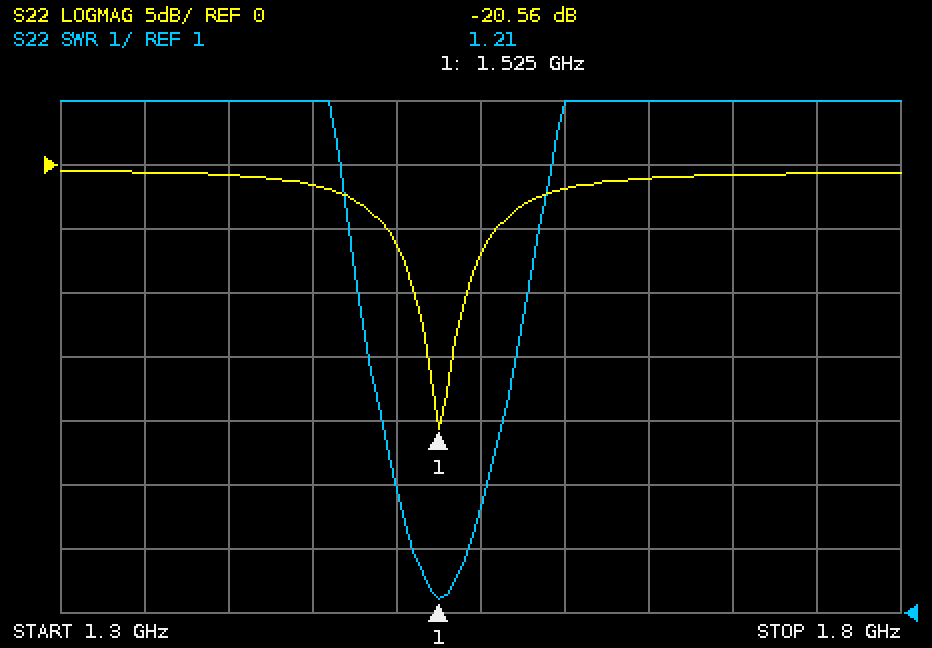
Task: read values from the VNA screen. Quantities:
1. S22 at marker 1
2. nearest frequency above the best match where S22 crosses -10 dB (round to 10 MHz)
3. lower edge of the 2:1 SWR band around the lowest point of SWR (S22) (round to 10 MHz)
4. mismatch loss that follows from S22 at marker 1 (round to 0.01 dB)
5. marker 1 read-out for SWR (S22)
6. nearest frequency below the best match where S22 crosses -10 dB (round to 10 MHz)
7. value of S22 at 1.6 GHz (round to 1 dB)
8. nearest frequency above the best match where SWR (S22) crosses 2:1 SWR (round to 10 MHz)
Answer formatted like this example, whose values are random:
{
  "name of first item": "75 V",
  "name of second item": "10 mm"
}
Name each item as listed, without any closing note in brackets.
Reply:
{
  "S22 at marker 1": "-20.56 dB",
  "nearest frequency above the best match where S22 crosses -10 dB": "1.54 GHz",
  "lower edge of the 2:1 SWR band around the lowest point of SWR (S22)": "1.51 GHz",
  "mismatch loss that follows from S22 at marker 1": "0.04 dB",
  "marker 1 read-out for SWR": "1.21",
  "nearest frequency below the best match where S22 crosses -10 dB": "1.51 GHz",
  "value of S22 at 1.6 GHz": "-2 dB",
  "nearest frequency above the best match where SWR (S22) crosses 2:1 SWR": "1.54 GHz"
}
